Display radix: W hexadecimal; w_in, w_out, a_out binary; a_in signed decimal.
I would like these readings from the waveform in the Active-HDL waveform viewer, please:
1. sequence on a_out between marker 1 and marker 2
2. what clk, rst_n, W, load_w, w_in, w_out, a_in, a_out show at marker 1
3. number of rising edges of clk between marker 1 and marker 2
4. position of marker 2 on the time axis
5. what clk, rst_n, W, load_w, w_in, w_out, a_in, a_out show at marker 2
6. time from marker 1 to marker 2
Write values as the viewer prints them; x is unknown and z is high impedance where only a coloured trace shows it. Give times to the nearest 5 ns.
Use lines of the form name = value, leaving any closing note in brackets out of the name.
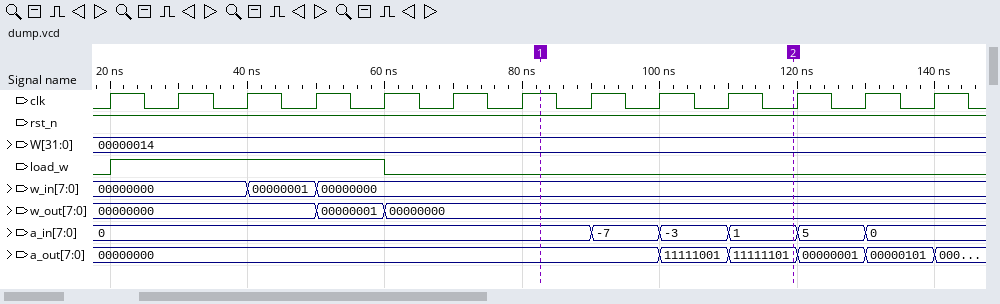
sequence on a_out between marker 1 and marker 2 = 00000000, 11111001, 11111101
what clk, rst_n, W, load_w, w_in, w_out, a_in, a_out show at marker 1 = clk=1, rst_n=1, W=00000014, load_w=0, w_in=00000000, w_out=00000000, a_in=0, a_out=00000000
number of rising edges of clk between marker 1 and marker 2 = 3
position of marker 2 on the time axis = 120 ns
what clk, rst_n, W, load_w, w_in, w_out, a_in, a_out show at marker 2 = clk=0, rst_n=1, W=00000014, load_w=0, w_in=00000000, w_out=00000000, a_in=1, a_out=11111101
time from marker 1 to marker 2 = 35 ns
